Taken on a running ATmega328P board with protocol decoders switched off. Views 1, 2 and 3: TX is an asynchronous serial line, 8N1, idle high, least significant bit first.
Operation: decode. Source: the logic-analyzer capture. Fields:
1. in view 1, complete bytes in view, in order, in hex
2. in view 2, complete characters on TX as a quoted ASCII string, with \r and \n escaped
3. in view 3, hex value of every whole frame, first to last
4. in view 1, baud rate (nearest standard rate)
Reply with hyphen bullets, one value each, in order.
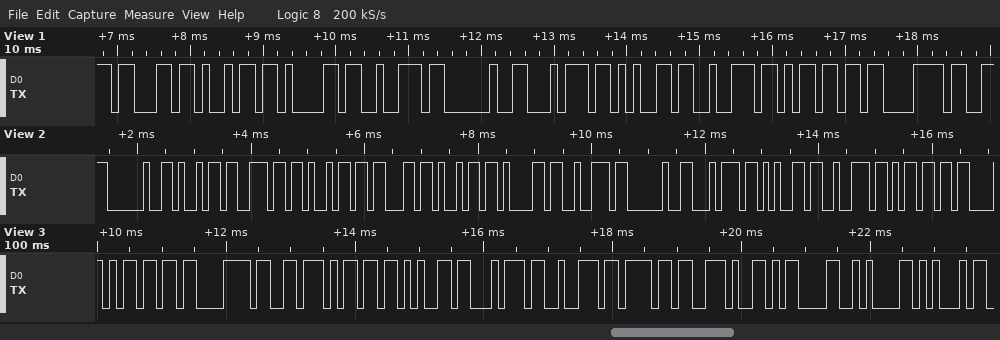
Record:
- 63 69 61 72 20 74 65 72 6D C3
- " iniciar term"
- 6D C3 B3 6D 65 74 72 6F 2E 0D 0A 45
- 9600 baud
